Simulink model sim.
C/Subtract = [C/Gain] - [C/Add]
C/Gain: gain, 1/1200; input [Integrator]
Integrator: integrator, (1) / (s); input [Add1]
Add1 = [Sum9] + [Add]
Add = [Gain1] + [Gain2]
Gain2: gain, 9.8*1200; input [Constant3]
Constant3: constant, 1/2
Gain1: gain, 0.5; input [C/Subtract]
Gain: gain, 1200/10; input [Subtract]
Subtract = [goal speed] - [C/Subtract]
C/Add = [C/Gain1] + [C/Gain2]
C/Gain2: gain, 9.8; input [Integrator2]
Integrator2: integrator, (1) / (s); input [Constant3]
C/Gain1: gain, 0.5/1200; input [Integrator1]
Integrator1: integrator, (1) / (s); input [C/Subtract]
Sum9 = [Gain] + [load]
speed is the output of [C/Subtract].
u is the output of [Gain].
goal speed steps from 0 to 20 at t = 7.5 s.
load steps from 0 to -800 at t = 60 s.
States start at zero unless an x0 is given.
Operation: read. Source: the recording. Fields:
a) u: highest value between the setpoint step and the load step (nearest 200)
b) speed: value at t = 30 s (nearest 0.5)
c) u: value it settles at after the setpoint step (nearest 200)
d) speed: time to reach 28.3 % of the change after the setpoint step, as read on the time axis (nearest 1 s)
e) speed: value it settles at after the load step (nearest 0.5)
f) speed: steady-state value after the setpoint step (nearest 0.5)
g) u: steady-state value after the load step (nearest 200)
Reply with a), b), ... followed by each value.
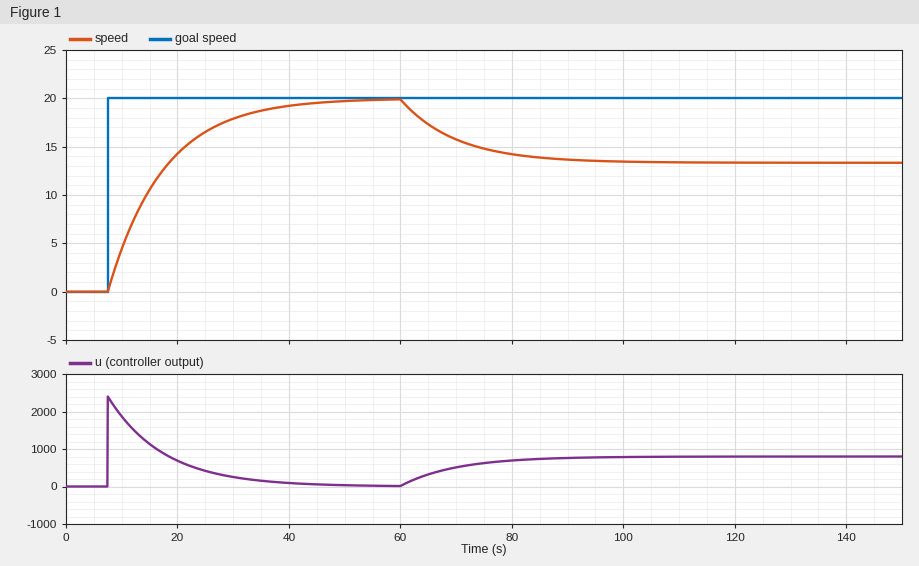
a) 2400
b) 18.0
c) 0
d) 11 s
e) 13.5
f) 20.0
g) 800
